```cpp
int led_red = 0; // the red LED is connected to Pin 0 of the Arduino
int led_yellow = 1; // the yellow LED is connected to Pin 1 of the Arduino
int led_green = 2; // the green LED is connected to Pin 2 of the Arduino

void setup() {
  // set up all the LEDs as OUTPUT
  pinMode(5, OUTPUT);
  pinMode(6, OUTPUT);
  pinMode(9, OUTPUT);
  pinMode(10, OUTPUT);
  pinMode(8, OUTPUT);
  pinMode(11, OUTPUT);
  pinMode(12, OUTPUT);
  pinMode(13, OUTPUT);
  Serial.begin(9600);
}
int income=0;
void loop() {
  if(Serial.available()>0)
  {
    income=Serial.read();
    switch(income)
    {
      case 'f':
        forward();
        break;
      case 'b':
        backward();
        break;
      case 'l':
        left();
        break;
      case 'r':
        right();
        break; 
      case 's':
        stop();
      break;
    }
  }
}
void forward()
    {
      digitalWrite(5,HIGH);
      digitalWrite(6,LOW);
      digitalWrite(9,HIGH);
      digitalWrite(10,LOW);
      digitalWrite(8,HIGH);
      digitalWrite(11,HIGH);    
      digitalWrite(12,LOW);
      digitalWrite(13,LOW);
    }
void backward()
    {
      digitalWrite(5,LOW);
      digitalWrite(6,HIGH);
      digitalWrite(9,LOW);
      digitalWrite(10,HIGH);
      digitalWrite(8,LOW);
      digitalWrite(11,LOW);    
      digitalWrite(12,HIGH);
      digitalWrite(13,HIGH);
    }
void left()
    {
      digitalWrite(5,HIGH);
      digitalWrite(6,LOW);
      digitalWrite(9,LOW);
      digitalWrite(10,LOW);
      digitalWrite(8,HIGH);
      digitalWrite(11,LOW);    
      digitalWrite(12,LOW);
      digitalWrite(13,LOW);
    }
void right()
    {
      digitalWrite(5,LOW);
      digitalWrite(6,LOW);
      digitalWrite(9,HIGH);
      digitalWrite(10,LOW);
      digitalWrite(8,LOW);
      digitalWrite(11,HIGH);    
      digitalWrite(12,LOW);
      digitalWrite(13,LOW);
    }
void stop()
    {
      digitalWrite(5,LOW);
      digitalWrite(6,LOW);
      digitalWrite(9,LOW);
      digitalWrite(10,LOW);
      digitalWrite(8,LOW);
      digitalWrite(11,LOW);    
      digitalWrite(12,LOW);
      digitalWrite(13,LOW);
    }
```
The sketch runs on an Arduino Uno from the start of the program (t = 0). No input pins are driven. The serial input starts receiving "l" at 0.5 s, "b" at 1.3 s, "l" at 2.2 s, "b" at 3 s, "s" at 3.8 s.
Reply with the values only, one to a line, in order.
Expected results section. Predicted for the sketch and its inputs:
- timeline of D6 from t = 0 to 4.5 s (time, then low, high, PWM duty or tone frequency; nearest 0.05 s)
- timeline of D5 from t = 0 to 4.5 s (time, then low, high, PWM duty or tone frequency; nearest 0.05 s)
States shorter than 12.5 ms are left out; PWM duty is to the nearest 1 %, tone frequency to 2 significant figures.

0 s low; 1.3 s high; 2.2 s low; 3 s high; 3.8 s low
0 s low; 0.5 s high; 1.3 s low; 2.2 s high; 3 s low
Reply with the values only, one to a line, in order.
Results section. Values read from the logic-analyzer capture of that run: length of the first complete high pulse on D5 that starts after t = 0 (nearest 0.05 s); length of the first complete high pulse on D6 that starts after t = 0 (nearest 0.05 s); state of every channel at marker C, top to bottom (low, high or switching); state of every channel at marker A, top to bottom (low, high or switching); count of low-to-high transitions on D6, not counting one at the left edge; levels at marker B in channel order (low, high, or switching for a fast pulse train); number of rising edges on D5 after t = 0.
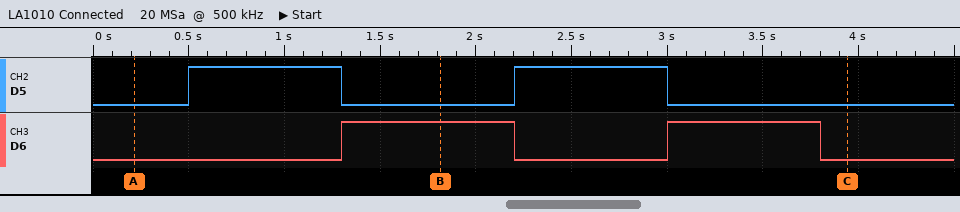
0.80 s
0.90 s
D5 low, D6 low
D5 low, D6 low
2
D5 low, D6 high
2
